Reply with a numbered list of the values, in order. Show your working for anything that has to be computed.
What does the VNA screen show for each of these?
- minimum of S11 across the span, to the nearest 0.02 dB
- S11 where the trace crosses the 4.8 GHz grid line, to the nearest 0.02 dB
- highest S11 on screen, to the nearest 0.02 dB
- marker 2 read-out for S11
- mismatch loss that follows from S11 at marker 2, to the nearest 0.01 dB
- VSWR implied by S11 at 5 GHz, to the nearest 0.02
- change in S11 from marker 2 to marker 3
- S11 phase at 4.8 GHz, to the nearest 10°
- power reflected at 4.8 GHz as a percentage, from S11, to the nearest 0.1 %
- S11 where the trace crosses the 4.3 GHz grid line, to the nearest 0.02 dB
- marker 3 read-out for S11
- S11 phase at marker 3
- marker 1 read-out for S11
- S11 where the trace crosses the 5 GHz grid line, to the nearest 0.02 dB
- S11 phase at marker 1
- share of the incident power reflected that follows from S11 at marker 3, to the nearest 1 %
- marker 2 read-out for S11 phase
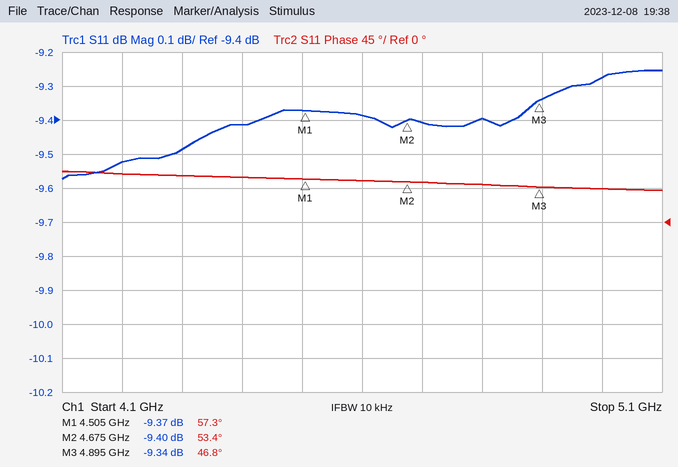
1. -9.58 dB
2. -9.40 dB
3. -9.26 dB
4. -9.40 dB
5. −10 log10(1 − 10^(-9.4/10)) ≈ 0.53 dB
6. |Γ| = 10^(-9.28/20) = 0.3436; VSWR = (1 + 0.3436)/(1 − 0.3436) ≈ 2.05, so 2.04 to the nearest 0.02
7. -9.34 − (-9.4) = 0.06 dB
8. 50°
9. 10^(-9.4/10) ≈ 11.5 %
10. -9.48 dB
11. -9.34 dB
12. 46.8°
13. -9.37 dB
14. -9.28 dB
15. 57.3°
16. 10^(-9.34/10) ≈ 12 %
17. 53.4°
